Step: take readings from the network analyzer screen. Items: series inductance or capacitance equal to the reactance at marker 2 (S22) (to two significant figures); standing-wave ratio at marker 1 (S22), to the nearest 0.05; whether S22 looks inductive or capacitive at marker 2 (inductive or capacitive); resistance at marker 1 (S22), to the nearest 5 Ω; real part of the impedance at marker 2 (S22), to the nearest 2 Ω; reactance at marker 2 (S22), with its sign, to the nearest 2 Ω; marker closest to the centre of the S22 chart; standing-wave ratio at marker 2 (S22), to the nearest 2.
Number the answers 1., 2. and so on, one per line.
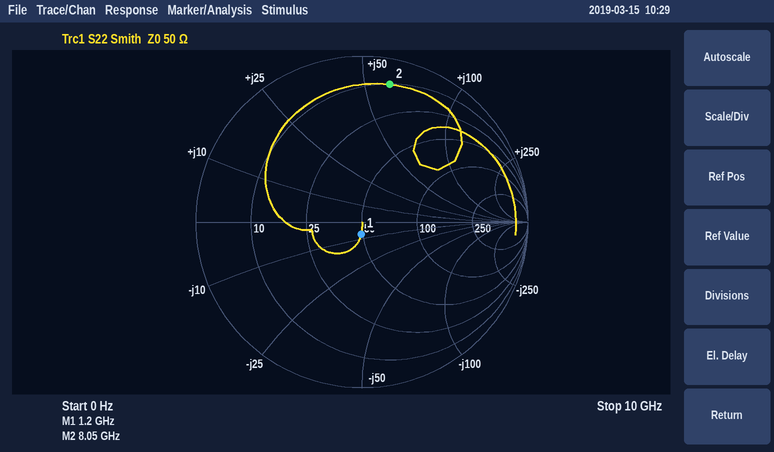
1. 1.2 nH
2. 1.15
3. inductive
4. 50 Ω
5. 10 Ω
6. +60 Ω
7. marker 1
8. 12
